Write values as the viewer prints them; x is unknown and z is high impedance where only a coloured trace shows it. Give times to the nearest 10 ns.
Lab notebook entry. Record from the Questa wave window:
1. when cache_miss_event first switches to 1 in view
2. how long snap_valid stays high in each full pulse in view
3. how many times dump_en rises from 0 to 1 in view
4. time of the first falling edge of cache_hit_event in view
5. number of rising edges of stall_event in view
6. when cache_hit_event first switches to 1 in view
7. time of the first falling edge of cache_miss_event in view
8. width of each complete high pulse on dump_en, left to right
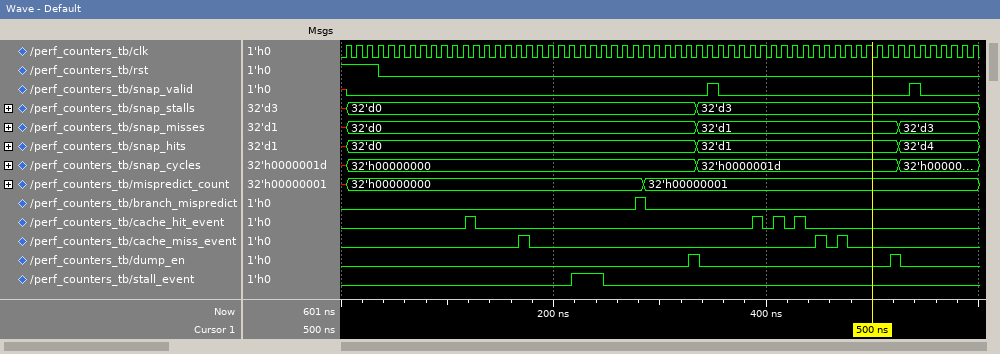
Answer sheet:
170 ns
10 ns, 10 ns
2
130 ns
1
120 ns
180 ns
10 ns, 10 ns
